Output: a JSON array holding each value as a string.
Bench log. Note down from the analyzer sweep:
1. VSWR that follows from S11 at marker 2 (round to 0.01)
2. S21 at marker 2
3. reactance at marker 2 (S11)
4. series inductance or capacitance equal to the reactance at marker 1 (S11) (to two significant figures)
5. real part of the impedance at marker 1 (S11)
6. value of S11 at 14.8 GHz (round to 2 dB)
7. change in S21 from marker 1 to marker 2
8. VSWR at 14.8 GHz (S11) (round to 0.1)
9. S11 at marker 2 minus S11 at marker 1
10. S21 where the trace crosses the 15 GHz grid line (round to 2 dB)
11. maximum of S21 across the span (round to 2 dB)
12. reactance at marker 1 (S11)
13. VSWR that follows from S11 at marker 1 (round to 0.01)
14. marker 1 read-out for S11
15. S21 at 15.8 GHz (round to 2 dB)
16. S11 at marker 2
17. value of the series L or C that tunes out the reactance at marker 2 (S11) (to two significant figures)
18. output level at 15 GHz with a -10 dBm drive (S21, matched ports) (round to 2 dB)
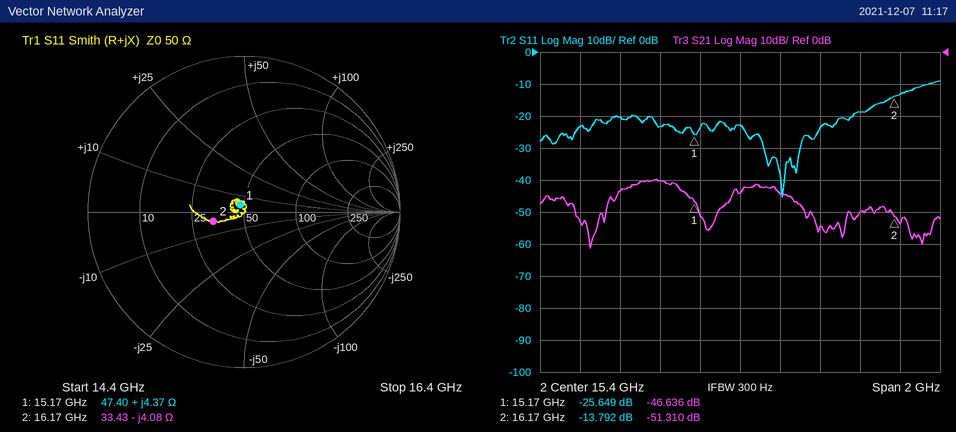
["1.51", "-51.310 dB", "-4.08 Ω", "46 pH", "47.40 Ω", "-20 dB", "-4.674 dB", "1.2", "11.857 dB", "-40 dB", "-40 dB", "+4.37 Ω", "1.11", "-25.649 dB", "-54 dB", "-13.792 dB", "40 pH", "-50 dBm"]
